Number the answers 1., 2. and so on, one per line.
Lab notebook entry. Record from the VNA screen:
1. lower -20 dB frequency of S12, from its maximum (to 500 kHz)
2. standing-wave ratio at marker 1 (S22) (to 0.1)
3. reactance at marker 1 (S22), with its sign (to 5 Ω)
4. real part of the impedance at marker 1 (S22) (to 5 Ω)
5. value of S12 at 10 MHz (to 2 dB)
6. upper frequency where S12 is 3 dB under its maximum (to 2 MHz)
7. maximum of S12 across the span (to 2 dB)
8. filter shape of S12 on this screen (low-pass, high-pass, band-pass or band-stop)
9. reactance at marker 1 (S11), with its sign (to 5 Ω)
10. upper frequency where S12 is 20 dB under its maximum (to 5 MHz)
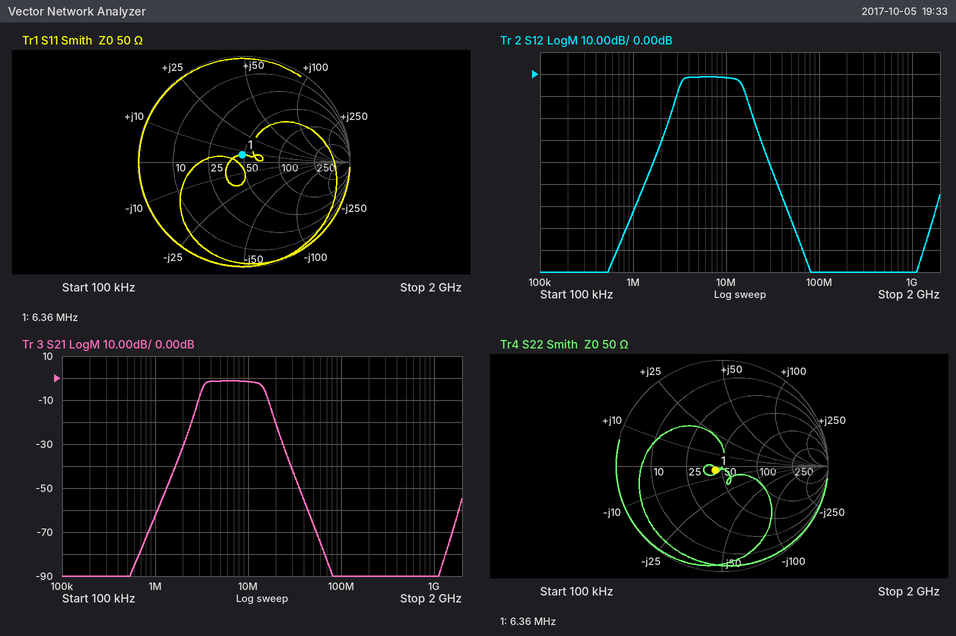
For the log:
1. 2.5 MHz
2. 1.2
3. -5 Ω
4. 45 Ω
5. -2 dB
6. 14 MHz
7. -2 dB
8. band-pass
9. +5 Ω
10. 20 MHz
